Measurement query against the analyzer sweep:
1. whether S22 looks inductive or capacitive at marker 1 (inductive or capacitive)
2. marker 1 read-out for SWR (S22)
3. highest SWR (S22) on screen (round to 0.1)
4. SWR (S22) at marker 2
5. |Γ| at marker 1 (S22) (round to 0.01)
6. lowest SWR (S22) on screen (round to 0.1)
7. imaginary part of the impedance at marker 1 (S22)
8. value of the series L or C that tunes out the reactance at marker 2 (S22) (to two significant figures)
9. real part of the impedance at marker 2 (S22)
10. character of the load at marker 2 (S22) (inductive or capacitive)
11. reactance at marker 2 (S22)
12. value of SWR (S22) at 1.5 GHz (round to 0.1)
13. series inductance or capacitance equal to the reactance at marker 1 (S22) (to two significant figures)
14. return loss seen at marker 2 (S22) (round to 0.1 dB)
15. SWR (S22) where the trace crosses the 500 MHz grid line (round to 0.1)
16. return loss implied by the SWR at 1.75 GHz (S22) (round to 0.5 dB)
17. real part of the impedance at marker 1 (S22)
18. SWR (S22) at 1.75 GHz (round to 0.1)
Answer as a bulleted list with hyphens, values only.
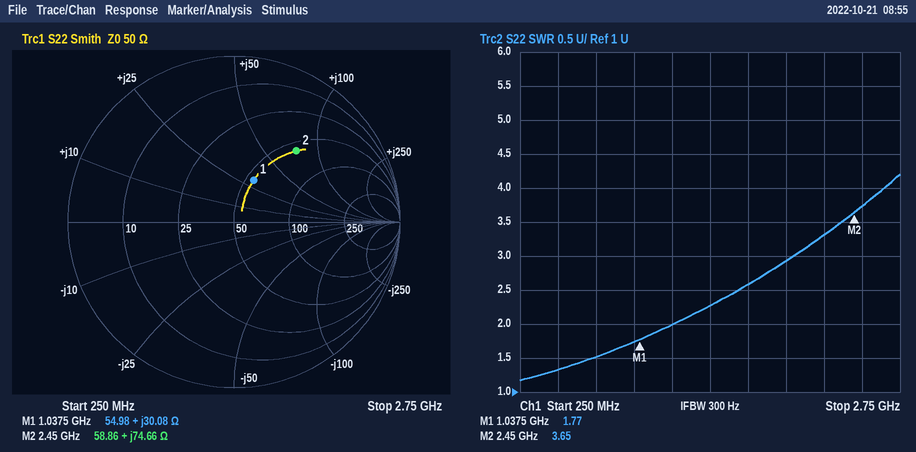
- inductive
- 1.77
- 4.2
- 3.65
- 0.28
- 1.2
- +30.08 Ω
- 870 fF
- 58.86 Ω
- inductive
- +74.66 Ω
- 2.3
- 4.6 nH
- 4.9 dB
- 1.3
- 7.0 dB
- 54.98 Ω
- 2.6
